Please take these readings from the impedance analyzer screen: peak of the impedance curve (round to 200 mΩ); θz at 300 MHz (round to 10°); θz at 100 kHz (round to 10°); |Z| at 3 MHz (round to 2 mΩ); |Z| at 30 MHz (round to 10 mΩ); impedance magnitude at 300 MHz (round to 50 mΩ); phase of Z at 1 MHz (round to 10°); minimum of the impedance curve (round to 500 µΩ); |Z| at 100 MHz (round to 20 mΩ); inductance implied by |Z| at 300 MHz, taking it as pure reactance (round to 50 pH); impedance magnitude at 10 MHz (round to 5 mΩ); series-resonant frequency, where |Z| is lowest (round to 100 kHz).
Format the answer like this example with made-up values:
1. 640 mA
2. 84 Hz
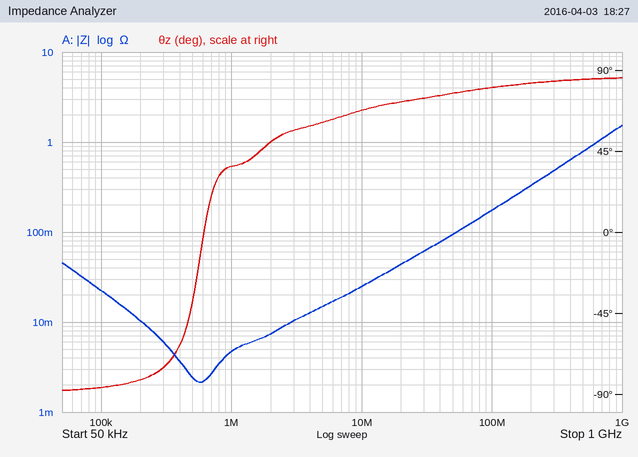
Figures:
1. 1.6 Ω
2. 80°
3. -90°
4. 10 mΩ
5. 60 mΩ
6. 500 mΩ
7. 40°
8. 2.0 mΩ
9. 180 mΩ
10. 250 pH
11. 25 mΩ
12. 600 kHz
